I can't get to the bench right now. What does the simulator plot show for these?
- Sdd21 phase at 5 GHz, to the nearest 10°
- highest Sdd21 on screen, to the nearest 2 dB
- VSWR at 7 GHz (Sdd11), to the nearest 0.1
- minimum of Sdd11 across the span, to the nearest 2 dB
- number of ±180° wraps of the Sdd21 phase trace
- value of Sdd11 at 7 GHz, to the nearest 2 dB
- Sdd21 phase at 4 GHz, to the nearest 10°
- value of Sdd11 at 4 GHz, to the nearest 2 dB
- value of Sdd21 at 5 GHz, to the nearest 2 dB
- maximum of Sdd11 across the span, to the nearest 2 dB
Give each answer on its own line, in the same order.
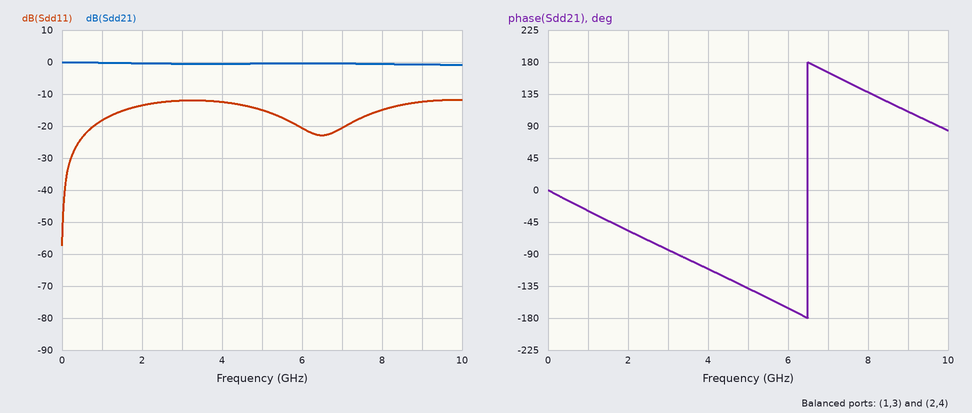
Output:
-140°
0 dB
1.2
-58 dB
1
-20 dB
-110°
-12 dB
0 dB
-12 dB
